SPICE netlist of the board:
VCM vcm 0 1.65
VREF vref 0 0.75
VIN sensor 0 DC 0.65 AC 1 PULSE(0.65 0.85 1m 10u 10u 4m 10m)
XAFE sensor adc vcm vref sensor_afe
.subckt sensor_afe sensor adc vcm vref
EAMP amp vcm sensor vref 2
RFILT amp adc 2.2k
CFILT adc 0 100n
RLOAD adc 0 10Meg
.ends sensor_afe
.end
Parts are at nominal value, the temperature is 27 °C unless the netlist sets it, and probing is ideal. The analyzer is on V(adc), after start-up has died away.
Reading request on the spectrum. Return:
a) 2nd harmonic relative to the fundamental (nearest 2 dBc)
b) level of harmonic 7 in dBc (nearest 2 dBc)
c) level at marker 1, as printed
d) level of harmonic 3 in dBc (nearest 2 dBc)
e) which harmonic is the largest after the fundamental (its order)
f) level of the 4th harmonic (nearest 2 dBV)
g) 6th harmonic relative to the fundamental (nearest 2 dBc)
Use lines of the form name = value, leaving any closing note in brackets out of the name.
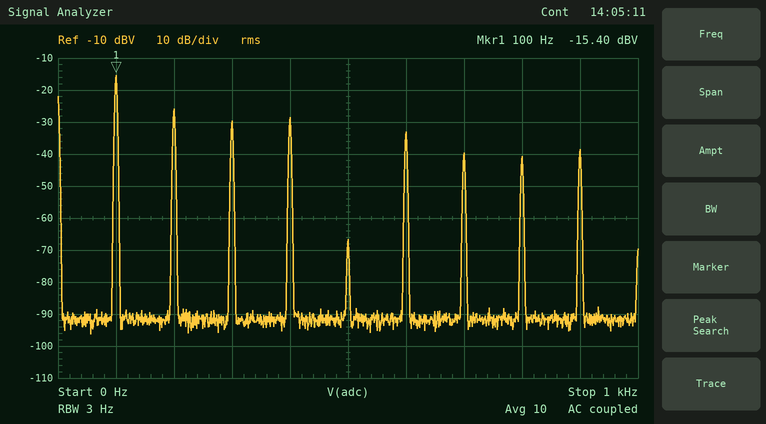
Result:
2nd harmonic relative to the fundamental = -10 dBc
level of harmonic 7 in dBc = -24 dBc
level at marker 1, as printed = -15.40 dBV
level of harmonic 3 in dBc = -14 dBc
which harmonic is the largest after the fundamental = 2
level of the 4th harmonic = -28 dBV
6th harmonic relative to the fundamental = -18 dBc
